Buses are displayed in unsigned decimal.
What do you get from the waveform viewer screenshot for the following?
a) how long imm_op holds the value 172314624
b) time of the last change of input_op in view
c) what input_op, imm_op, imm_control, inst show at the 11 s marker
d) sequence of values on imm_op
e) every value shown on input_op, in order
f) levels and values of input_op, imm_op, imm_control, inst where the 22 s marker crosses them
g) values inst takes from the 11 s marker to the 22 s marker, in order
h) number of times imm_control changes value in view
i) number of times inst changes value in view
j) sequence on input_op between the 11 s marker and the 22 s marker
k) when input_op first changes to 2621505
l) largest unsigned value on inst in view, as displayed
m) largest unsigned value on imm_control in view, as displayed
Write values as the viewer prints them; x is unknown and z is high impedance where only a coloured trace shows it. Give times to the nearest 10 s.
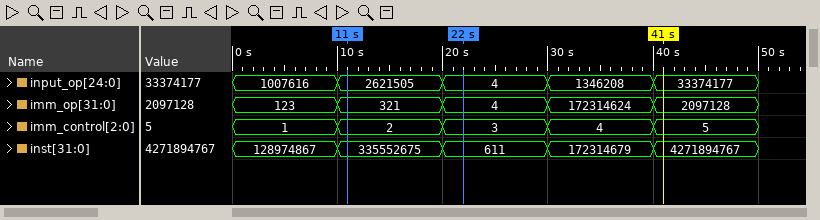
10 s
40 s
input_op=2621505, imm_op=321, imm_control=2, inst=335552675
123, 321, 4, 172314624, 2097128
1007616, 2621505, 4, 1346208, 33374177
input_op=4, imm_op=4, imm_control=3, inst=611
335552675, 611
4
4
2621505, 4
10 s
4271894767
5
